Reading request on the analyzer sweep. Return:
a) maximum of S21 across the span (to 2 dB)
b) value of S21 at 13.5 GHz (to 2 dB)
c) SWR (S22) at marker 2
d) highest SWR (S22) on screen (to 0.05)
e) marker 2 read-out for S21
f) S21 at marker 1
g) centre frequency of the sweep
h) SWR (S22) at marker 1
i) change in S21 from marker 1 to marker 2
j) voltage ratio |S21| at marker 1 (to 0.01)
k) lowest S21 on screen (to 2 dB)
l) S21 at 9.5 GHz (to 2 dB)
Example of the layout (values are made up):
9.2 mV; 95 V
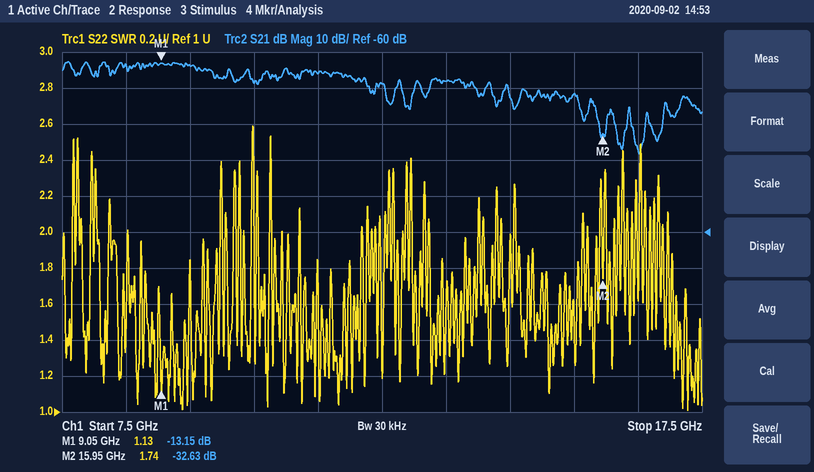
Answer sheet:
-12 dB; -18 dB; 1.74; 2.60; -32.63 dB; -13.15 dB; 12.5 GHz; 1.13; -19.48 dB; 0.22; -38 dB; -14 dB
